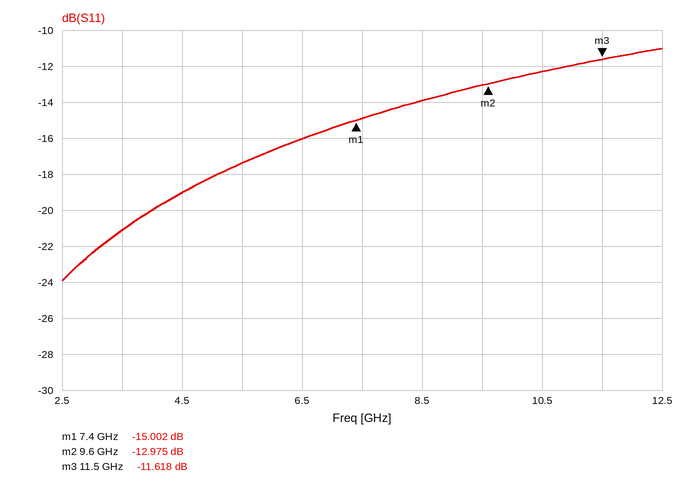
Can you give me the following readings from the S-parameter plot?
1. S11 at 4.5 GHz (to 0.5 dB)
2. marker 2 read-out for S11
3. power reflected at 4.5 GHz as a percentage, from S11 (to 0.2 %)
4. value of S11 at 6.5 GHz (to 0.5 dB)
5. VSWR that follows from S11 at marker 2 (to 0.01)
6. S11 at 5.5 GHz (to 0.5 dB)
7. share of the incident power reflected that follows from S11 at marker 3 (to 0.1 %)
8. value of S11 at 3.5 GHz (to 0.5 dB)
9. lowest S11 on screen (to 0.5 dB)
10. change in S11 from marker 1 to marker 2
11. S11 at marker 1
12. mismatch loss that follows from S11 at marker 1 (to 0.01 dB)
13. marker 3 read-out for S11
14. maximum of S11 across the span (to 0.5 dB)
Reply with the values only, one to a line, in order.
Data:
-19.0 dB
-12.975 dB
1.2 %
-16.0 dB
1.58
-17.5 dB
6.9 %
-21.0 dB
-24.0 dB
2.027 dB
-15.002 dB
0.14 dB
-11.618 dB
-11.0 dB
